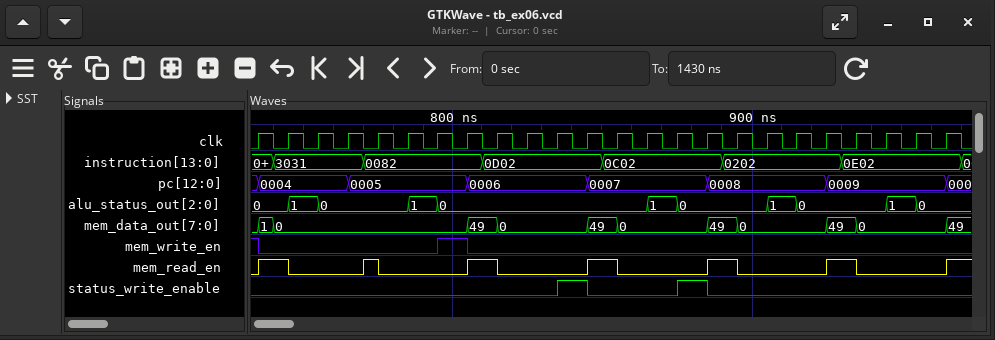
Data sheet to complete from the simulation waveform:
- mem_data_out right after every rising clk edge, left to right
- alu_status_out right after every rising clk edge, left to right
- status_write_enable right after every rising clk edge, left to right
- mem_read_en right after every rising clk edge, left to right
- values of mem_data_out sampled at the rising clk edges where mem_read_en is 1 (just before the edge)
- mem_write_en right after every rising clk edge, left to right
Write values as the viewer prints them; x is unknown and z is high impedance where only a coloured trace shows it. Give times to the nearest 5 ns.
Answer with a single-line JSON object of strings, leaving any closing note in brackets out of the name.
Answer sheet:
{"mem_data_out right after every rising clk edge, left to right": "1, 0, 0, 0, 0, 0, 0, 49, 0, 0, 0, 49, 0, 0, 0, 49, 0, 0, 0, 49, 0, 0, 0, 49", "alu_status_out right after every rising clk edge, left to right": "0, 1, 0, 0, 0, 1, 0, 0, 0, 0, 0, 0, 0, 1, 0, 0, 0, 1, 0, 0, 0, 1, 0, 0", "status_write_enable right after every rising clk edge, left to right": "0 0 0 0 0 0 0 0 0 0 1 0 0 0 1 0 0 0 0 0 0 0 0 0", "mem_read_en right after every rising clk edge, left to right": "1 0 0 0 0 0 0 1 0 0 0 1 0 0 0 1 0 0 0 1 0 0 0 1", "values of mem_data_out sampled at the rising clk edges where mem_read_en is 1": "0, 0, 49, 49, 49, 49", "mem_write_en right after every rising clk edge, left to right": "0 0 0 0 0 0 1 0 0 0 0 0 0 0 0 0 0 0 0 0 0 0 0 0"}
